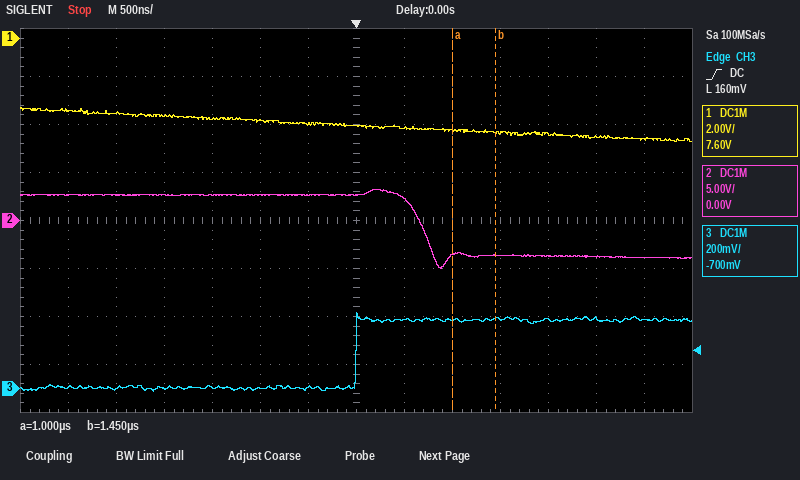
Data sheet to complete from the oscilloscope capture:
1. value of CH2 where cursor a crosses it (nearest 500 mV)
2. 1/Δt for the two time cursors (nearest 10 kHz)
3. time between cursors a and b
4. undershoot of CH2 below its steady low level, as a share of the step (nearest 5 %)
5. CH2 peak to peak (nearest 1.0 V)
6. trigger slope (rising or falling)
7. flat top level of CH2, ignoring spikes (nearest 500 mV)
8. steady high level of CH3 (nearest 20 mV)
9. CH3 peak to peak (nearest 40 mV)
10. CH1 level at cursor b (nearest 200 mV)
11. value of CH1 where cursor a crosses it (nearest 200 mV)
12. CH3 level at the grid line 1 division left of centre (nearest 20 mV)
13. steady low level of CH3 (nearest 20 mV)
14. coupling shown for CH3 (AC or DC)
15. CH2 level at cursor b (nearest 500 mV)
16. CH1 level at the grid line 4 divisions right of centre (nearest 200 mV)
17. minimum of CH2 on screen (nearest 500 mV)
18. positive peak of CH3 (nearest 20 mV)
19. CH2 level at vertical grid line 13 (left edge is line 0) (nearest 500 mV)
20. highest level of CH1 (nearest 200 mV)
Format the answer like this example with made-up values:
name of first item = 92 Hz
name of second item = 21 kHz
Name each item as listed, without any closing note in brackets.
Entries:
value of CH2 where cursor a crosses it = -3.5 V
1/Δt for the two time cursors = 2.22 MHz
time between cursors a and b = 450 ns
undershoot of CH2 below its steady low level, as a share of the step = 20 %
CH2 peak to peak = 8.0 V
trigger slope = rising
flat top level of CH2, ignoring spikes = 2.5 V
steady high level of CH3 = 280 mV
CH3 peak to peak = 320 mV
CH1 level at cursor b = -4.0 V
value of CH1 where cursor a crosses it = -3.8 V
CH3 level at the grid line 1 division left of centre = 0 mV
steady low level of CH3 = 0 mV
coupling shown for CH3 = DC
CH2 level at cursor b = -3.5 V
CH1 level at the grid line 4 divisions right of centre = -4.0 V
minimum of CH2 on screen = -5.0 V
positive peak of CH3 = 320 mV
CH2 level at vertical grid line 13 (left edge is line 0) = -4.0 V
highest level of CH1 = -2.8 V
